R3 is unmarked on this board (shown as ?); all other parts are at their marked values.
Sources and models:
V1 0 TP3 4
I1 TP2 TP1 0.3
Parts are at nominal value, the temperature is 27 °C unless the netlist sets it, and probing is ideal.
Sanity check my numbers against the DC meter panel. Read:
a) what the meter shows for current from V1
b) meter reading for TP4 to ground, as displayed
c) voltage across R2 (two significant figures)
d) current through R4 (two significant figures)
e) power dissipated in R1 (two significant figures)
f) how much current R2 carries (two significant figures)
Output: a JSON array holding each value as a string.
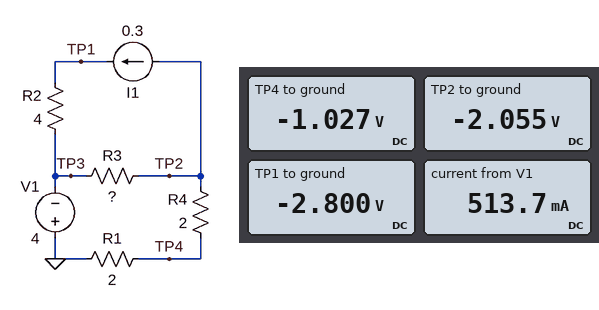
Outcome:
["513.7 mA", "-1.027 V", "1.2 V", "510 mA", "530 mW", "300 mA"]
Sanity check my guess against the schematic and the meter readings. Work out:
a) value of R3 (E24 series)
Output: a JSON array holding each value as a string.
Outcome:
["9.1 Ω"]
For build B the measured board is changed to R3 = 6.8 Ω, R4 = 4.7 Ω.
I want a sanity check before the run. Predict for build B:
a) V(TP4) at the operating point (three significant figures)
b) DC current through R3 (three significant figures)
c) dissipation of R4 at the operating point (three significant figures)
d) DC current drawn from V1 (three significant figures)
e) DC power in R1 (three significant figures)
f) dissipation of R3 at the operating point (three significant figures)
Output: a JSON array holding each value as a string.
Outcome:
["-895 mV", "147 mA", "941 mW", "447 mA", "400 mW", "148 mW"]
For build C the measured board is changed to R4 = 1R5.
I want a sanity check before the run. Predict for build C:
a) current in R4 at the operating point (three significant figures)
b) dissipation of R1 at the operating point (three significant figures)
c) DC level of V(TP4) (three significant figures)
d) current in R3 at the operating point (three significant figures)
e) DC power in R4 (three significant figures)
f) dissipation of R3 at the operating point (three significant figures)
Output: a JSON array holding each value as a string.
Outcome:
["534 mA", "571 mW", "-1.07 V", "234 mA", "428 mW", "499 mW"]
